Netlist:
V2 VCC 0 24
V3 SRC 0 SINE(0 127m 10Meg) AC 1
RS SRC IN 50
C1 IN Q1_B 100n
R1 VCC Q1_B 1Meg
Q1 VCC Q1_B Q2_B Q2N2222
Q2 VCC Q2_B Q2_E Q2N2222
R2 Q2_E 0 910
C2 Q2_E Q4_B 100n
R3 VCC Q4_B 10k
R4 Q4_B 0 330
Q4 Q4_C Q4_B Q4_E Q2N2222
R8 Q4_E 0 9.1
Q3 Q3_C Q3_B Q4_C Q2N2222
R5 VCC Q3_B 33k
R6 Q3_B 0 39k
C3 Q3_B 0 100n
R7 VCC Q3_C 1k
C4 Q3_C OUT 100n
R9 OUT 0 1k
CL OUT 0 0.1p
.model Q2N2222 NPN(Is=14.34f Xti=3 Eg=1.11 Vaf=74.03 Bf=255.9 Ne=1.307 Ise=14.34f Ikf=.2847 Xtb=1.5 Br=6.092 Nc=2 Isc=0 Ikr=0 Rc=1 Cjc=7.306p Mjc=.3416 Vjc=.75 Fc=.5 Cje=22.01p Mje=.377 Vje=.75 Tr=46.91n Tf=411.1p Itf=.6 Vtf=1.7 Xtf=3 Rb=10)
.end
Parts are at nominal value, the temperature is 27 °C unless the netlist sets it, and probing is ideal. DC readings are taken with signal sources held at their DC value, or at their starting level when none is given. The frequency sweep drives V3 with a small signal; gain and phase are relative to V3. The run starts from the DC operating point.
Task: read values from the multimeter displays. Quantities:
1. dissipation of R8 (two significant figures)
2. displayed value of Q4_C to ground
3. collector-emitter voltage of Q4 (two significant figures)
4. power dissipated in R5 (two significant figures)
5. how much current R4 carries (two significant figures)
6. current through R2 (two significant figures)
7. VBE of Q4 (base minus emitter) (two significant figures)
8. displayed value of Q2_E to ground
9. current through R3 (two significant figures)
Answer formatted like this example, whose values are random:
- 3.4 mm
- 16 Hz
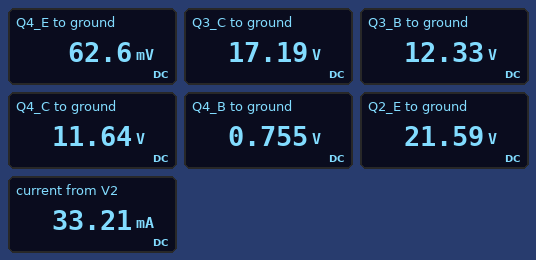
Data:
- 430 µW
- 11.64 V
- 12 V
- 4.1 mW
- 2.3 mA
- 24 mA
- 690 mV
- 21.59 V
- 2.3 mA
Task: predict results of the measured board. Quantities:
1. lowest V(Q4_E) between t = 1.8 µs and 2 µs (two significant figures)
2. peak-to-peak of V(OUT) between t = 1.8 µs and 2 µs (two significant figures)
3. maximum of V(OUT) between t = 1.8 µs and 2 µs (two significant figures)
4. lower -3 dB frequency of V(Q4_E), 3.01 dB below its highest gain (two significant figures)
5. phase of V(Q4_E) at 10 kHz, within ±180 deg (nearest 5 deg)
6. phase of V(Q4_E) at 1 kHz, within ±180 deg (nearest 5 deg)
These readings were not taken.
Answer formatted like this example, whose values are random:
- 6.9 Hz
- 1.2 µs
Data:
- 5.0 mV
- 8.3 V
- 3.1 V
- 5.5 kHz
- 30 deg
- 80 deg
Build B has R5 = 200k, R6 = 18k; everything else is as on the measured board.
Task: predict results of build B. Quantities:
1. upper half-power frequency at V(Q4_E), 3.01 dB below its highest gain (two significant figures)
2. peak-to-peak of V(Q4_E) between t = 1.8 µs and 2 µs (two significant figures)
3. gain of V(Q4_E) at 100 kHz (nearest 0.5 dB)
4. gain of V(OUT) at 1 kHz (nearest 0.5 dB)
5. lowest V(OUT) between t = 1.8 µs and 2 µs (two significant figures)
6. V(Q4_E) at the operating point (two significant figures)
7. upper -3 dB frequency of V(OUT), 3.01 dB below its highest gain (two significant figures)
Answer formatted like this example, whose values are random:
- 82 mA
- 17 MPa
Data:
- 88 MHz
- 150 mV
- -3.5 dB
- 14.0 dB
- -5.3 V
- 59 mV
- 67 MHz
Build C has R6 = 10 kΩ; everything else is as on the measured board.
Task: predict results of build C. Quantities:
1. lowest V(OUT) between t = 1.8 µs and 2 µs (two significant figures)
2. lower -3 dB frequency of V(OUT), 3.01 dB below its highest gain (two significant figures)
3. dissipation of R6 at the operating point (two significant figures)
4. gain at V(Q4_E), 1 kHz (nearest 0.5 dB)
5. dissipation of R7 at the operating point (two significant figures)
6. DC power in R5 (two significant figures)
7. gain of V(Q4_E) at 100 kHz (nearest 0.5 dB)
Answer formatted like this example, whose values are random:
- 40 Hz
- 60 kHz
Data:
- -5.3 V
- 5.7 kHz
- 2.8 mW
- -18.5 dB
- 43 mW
- 11 mW
- -3.5 dB
